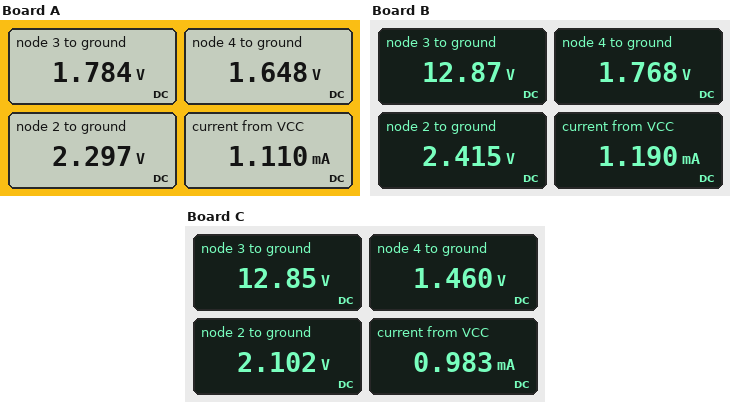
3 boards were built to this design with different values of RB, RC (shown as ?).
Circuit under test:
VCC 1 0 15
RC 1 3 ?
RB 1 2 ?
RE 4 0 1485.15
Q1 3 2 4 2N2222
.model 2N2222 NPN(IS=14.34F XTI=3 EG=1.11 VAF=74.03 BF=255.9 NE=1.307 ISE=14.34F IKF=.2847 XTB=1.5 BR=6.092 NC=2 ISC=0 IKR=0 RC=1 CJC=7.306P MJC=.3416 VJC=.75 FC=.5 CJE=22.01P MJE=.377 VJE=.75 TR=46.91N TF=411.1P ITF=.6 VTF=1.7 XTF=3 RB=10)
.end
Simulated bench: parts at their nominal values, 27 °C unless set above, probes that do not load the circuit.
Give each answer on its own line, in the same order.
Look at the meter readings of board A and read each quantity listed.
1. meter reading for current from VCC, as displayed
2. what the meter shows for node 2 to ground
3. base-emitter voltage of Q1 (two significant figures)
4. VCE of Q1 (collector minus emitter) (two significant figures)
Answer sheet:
1.110 mA
2.297 V
650 mV
140 mV
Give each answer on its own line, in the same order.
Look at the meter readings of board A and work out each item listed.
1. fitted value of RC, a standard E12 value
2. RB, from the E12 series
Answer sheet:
12 kΩ
1.5 MΩ
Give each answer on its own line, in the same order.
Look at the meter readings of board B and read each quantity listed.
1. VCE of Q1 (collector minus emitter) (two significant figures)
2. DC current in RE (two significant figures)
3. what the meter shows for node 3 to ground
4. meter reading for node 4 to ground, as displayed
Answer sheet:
11 V
1.2 mA
12.87 V
1.768 V
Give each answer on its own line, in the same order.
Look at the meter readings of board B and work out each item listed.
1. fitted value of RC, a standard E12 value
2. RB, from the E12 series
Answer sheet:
1.8 kΩ
1.8 MΩ
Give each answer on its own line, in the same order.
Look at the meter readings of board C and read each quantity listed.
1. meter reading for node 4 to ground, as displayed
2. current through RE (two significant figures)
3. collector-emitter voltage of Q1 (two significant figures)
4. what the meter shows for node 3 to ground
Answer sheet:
1.460 V
980 µA
11 V
12.85 V
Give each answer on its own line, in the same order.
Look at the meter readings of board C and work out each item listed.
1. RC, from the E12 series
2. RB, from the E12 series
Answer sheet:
2.2 kΩ
2.2 MΩ
